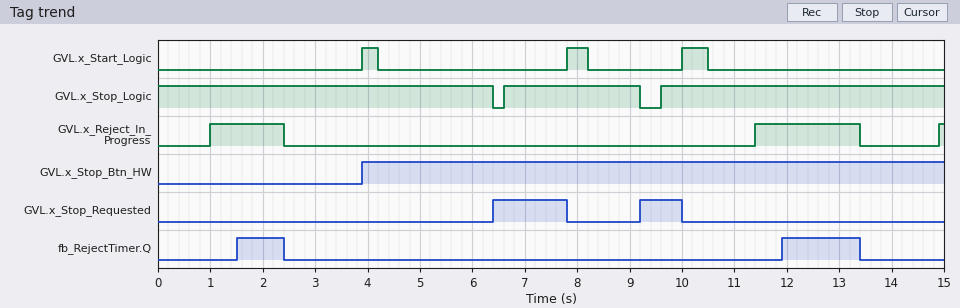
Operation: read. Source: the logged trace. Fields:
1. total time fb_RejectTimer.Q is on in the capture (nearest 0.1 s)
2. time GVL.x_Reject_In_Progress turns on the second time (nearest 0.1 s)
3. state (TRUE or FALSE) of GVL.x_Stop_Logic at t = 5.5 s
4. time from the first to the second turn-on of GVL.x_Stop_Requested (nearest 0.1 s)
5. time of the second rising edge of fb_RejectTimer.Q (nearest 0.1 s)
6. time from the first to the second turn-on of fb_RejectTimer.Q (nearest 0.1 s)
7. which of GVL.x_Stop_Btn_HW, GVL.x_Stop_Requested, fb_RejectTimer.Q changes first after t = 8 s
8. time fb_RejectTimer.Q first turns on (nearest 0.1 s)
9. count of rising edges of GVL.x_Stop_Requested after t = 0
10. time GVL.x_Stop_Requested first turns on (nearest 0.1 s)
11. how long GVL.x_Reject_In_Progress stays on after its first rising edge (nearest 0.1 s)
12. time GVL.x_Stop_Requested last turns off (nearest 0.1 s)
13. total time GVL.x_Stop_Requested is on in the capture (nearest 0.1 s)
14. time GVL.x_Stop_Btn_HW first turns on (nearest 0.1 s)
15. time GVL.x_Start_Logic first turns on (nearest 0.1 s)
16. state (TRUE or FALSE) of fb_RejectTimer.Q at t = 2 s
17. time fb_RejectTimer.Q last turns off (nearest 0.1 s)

2.4 s
11.4 s
TRUE
2.8 s
11.9 s
10.4 s
GVL.x_Stop_Requested
1.5 s
2
6.4 s
1.4 s
10.0 s
2.2 s
3.9 s
3.9 s
TRUE
13.4 s
